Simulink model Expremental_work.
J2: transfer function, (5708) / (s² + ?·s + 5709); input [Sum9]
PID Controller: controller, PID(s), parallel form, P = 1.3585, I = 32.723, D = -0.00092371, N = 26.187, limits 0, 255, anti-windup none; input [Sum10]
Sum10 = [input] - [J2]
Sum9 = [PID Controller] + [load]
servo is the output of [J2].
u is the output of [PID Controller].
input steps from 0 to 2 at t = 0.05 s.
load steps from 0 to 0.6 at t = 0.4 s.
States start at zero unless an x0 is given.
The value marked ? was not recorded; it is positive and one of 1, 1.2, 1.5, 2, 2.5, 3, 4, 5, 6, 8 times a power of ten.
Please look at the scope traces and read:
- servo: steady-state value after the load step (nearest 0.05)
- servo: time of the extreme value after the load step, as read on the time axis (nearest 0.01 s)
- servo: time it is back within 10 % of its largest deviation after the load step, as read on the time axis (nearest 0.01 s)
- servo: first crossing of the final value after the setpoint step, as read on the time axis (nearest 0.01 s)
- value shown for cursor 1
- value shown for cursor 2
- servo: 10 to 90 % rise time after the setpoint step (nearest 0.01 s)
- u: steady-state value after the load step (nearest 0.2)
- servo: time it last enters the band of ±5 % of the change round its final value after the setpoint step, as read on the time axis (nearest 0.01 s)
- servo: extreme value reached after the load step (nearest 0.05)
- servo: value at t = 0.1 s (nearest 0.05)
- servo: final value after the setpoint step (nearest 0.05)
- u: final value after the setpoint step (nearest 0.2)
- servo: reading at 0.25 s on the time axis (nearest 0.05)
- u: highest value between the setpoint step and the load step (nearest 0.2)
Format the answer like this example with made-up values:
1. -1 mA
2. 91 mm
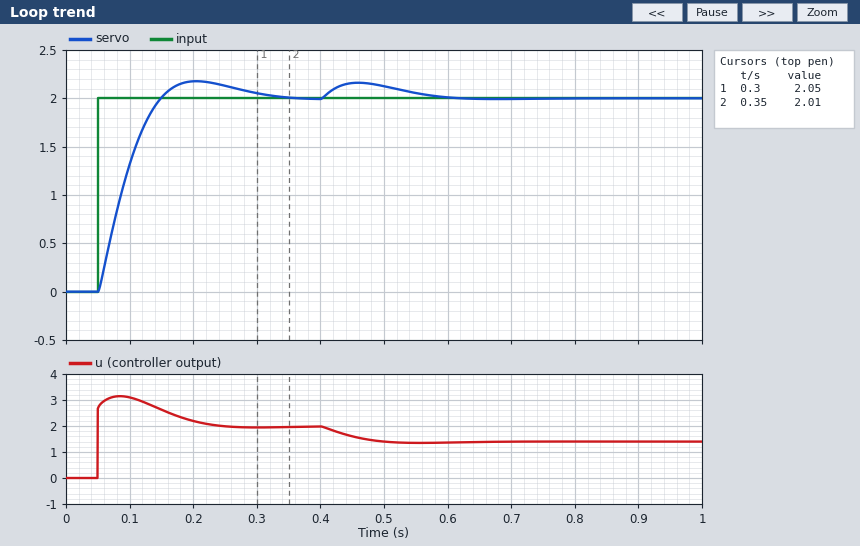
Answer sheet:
1. 2.00
2. 0.46 s
3. 0.59 s
4. 0.15 s
5. 2.05
6. 2.01
7. 0.07 s
8. 1.4
9. 0.27 s
10. 2.15
11. 1.30
12. 2.00
13. 2.0
14. 2.15
15. 3.2
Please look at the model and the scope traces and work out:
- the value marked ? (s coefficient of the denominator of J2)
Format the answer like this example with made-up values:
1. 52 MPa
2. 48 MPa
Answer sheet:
1. 500
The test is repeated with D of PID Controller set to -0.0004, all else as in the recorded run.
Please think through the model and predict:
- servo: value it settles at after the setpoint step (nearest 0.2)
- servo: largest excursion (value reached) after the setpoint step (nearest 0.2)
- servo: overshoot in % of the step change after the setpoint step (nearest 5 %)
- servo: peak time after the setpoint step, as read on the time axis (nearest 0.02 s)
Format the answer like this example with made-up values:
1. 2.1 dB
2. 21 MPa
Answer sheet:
1. 2.0
2. 2.2
3. 10 %
4. 0.20 s
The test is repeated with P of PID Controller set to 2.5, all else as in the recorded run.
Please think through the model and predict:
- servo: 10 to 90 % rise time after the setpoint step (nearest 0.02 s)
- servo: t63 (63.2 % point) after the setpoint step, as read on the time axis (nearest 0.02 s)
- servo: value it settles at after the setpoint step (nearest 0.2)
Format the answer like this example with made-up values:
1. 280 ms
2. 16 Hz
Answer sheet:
1. 0.06 s
2. 0.08 s
3. 2.0
